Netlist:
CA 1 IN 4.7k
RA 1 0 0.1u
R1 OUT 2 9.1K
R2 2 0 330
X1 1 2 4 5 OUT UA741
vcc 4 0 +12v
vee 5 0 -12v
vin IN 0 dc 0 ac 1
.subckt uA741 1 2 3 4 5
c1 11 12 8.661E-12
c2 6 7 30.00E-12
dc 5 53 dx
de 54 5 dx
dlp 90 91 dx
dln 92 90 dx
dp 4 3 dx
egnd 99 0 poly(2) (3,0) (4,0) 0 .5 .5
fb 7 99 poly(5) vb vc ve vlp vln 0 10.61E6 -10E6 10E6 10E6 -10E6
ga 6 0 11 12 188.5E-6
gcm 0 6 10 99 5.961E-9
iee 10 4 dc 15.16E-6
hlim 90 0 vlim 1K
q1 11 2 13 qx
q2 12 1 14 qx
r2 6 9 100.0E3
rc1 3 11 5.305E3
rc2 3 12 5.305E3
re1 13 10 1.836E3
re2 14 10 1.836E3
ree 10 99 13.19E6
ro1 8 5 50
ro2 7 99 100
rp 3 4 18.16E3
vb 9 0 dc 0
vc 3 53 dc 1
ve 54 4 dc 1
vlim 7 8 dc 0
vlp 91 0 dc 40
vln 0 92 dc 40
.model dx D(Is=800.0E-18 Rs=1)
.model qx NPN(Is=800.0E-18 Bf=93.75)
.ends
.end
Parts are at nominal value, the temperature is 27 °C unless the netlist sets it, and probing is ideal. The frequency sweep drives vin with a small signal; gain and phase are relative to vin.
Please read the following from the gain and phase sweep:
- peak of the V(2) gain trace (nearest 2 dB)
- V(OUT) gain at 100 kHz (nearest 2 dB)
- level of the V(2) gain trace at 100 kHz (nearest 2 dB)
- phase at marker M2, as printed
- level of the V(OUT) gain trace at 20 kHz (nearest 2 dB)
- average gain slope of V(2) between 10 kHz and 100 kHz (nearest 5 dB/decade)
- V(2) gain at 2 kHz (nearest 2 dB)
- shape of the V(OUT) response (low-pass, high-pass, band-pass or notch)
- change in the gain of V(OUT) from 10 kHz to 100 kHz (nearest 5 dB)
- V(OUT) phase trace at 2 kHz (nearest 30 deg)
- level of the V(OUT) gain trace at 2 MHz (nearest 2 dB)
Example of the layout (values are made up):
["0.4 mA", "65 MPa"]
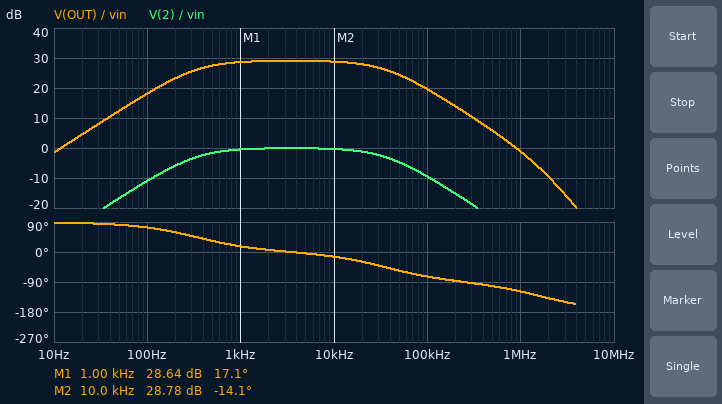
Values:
["0 dB", "20 dB", "-10 dB", "-14.1 deg", "28 dB", "-10 dB/decade", "0 dB", "band-pass", "-10 dB", "0 deg", "-10 dB"]
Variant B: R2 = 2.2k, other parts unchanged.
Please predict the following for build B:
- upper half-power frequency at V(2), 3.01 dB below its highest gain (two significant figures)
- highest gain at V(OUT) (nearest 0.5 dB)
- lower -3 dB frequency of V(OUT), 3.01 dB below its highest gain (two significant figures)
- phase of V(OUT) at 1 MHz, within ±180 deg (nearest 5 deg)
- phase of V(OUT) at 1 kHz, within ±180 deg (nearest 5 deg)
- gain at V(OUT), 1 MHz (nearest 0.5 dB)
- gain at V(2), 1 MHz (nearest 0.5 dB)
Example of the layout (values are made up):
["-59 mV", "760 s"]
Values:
["220 kHz", "14.0 dB", "340 Hz", "-110 deg", "20 deg", "-0.5 dB", "-15.0 dB"]
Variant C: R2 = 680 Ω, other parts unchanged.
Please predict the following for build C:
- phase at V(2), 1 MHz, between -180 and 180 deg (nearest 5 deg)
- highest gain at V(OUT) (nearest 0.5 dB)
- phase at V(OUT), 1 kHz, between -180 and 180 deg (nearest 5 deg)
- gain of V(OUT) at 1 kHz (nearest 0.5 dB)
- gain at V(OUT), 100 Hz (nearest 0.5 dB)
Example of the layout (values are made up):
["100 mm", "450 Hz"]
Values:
["-115 deg", "23.0 dB", "20 deg", "22.5 dB", "12.0 dB"]
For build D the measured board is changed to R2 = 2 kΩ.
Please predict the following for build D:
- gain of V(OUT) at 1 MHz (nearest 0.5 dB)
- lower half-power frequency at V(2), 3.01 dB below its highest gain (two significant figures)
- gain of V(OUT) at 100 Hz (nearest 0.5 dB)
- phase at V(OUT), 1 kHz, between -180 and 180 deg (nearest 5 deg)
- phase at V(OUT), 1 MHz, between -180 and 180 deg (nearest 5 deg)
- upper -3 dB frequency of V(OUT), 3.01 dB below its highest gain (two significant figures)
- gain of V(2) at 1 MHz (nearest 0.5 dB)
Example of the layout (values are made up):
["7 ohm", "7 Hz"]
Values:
["-0.5 dB", "340 Hz", "4.0 dB", "20 deg", "-110 deg", "200 kHz", "-15.5 dB"]
